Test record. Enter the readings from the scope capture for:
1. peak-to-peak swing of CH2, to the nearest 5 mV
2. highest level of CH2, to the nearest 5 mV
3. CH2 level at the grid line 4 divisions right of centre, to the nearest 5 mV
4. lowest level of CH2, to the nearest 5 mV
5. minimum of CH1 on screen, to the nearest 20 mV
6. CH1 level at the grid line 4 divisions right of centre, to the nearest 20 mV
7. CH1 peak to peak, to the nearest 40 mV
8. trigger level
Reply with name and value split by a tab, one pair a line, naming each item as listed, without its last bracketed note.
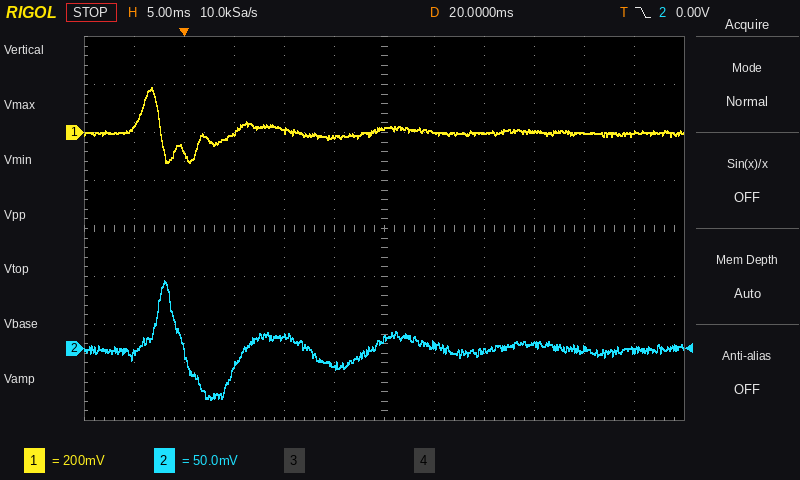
peak-to-peak swing of CH2, to the nearest 5 mV	125 mV
highest level of CH2, to the nearest 5 mV	70 mV
CH2 level at the grid line 4 divisions right of centre, to the nearest 5 mV	0 mV
lowest level of CH2, to the nearest 5 mV	-55 mV
minimum of CH1 on screen, to the nearest 20 mV	-120 mV
CH1 level at the grid line 4 divisions right of centre, to the nearest 20 mV	0 mV
CH1 peak to peak, to the nearest 40 mV	320 mV
trigger level	0.00 V
